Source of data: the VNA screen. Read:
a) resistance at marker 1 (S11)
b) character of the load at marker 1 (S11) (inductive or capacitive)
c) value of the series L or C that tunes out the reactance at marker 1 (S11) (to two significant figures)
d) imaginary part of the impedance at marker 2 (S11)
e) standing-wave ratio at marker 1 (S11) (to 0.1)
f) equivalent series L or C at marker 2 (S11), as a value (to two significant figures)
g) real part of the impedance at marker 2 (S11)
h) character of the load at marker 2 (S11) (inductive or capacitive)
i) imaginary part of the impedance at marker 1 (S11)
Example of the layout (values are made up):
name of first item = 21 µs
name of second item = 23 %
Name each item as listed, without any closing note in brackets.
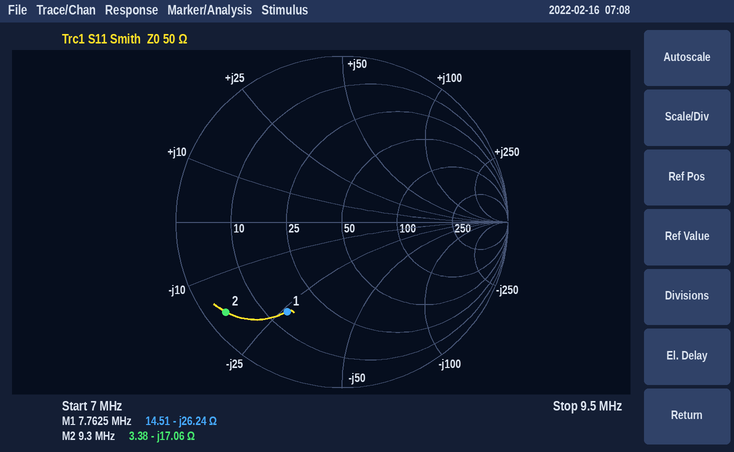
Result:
resistance at marker 1 = 14.51 Ω
character of the load at marker 1 (S11) = capacitive
value of the series L or C that tunes out the reactance at marker 1 (S11) = 540 nH
imaginary part of the impedance at marker 2 = -17.06 Ω
standing-wave ratio at marker 1 (S11) = 4.5
equivalent series L or C at marker 2 (S11), as a value = 1.0 nF
real part of the impedance at marker 2 = 3.38 Ω
character of the load at marker 2 (S11) = capacitive
imaginary part of the impedance at marker 1 = -26.24 Ω
